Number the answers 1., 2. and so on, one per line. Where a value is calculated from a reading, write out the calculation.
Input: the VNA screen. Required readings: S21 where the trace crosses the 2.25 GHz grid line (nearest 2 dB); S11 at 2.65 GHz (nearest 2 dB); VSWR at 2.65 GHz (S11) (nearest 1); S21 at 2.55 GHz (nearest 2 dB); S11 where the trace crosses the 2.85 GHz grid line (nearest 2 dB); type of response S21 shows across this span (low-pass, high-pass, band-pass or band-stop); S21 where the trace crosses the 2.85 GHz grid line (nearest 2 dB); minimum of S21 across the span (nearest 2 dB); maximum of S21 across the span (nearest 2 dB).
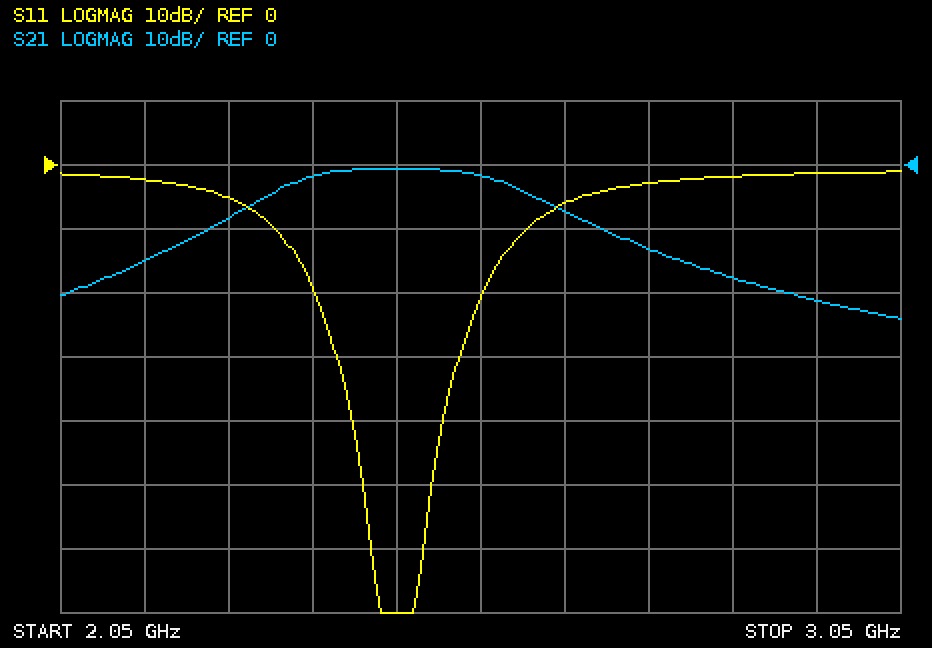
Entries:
1. -8 dB
2. -6 dB
3. |Γ| = 10^(-6/20) = 0.5012; VSWR = (1 + 0.5012)/(1 − 0.5012) ≈ 3
4. -2 dB
5. -2 dB
6. band-pass
7. -18 dB
8. -24 dB
9. 0 dB
